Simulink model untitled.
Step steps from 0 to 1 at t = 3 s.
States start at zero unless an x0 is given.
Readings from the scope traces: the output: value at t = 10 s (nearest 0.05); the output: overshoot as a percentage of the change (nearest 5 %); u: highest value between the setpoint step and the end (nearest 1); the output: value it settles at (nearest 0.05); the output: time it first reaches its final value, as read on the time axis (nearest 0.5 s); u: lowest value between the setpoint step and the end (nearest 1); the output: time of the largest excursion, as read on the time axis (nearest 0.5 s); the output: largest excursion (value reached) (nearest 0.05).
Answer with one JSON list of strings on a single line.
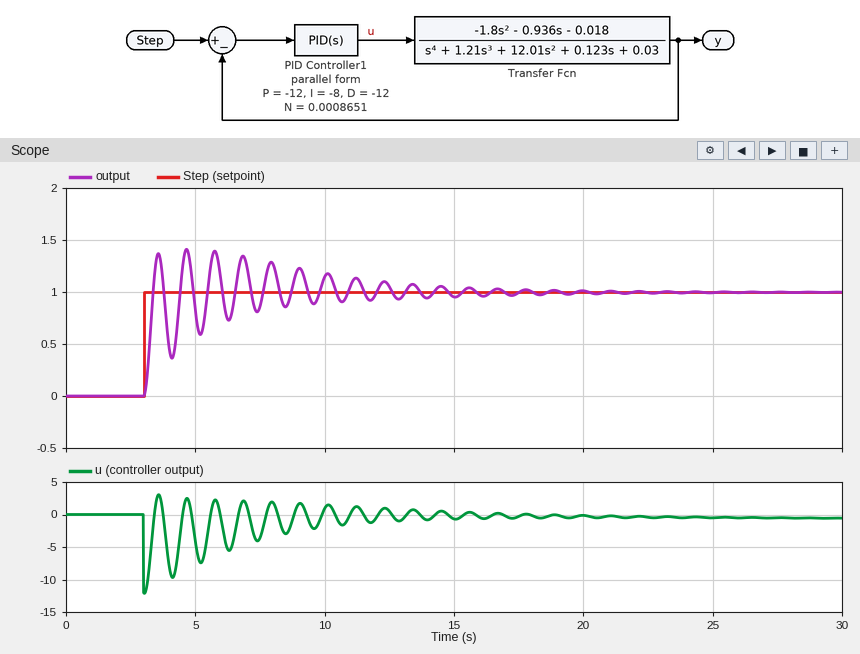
["1.15", "40 %", "3", "1.00", "3.5 s", "-12", "4.5 s", "1.40"]
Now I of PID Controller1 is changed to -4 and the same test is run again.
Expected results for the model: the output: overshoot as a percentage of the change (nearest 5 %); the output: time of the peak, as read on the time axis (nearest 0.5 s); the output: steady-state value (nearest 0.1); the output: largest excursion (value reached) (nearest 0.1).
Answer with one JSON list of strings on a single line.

["30 %", "3.5 s", "1.0", "1.3"]
